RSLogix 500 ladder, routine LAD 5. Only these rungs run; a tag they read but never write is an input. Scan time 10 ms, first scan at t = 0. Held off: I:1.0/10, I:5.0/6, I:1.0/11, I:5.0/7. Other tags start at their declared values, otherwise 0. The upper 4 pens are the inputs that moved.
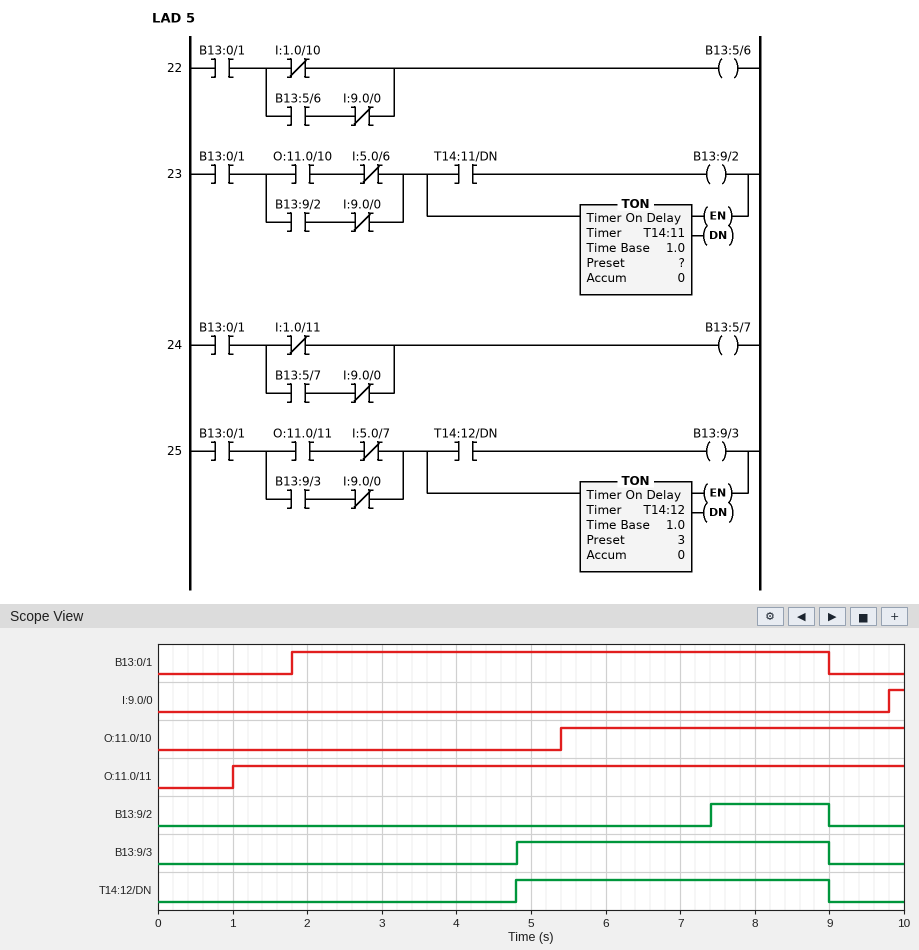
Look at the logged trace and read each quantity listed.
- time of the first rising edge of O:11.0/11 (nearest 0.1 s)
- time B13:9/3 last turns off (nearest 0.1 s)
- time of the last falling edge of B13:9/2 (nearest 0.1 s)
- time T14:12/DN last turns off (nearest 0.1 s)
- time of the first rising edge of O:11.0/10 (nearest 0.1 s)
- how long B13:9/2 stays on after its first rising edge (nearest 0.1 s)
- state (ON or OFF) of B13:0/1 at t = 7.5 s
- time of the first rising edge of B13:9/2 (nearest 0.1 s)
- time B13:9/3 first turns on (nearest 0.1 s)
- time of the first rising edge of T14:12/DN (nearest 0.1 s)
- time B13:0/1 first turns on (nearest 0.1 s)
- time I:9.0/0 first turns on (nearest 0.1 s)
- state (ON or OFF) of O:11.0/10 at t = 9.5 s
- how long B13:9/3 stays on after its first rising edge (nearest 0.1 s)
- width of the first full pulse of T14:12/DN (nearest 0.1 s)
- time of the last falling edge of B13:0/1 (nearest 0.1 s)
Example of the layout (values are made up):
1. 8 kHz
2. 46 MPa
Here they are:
1. 1.0 s
2. 9.0 s
3. 9.0 s
4. 9.0 s
5. 5.4 s
6. 1.6 s
7. ON
8. 7.4 s
9. 4.8 s
10. 4.8 s
11. 1.8 s
12. 9.8 s
13. ON
14. 4.2 s
15. 4.2 s
16. 9.0 s
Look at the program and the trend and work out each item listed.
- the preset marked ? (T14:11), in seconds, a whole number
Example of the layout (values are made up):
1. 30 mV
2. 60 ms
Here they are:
1. 2 s
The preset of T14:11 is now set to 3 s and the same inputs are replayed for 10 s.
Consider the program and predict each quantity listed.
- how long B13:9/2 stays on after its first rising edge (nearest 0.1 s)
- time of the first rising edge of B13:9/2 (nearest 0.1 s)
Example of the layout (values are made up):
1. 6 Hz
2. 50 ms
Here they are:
1. 0.6 s
2. 8.4 s
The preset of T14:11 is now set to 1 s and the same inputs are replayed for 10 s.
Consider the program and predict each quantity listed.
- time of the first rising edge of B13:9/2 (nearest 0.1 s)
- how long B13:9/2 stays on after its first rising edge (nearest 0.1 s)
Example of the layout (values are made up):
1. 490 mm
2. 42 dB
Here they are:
1. 6.4 s
2. 2.6 s
